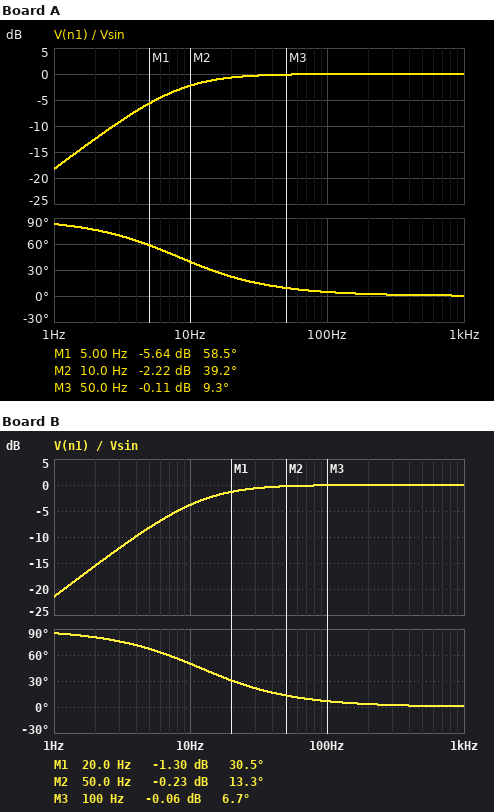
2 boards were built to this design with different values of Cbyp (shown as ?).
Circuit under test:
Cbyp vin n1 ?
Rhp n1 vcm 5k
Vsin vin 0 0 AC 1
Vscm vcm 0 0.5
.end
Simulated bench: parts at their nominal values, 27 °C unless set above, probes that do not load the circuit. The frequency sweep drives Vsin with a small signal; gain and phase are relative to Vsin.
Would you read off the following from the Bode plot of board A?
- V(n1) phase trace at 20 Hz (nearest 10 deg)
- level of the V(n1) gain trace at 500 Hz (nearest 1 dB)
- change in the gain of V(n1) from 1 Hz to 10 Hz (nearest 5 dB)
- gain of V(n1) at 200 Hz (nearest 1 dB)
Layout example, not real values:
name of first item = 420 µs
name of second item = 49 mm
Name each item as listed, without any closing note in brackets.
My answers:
V(n1) phase trace at 20 Hz = 20 deg
level of the V(n1) gain trace at 500 Hz = 0 dB
change in the gain of V(n1) from 1 Hz to 10 Hz = 15 dB
gain of V(n1) at 200 Hz = 0 dB
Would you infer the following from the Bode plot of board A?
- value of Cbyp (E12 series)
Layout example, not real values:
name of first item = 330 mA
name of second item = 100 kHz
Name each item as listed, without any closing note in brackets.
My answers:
value of Cbyp = 3.9 µF
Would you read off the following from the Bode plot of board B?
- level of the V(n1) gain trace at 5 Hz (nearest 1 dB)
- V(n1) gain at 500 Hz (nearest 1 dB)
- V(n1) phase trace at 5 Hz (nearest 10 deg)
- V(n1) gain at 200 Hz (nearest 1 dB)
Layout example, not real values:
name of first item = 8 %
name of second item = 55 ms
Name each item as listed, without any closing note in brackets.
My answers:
level of the V(n1) gain trace at 5 Hz = -8 dB
V(n1) gain at 500 Hz = 0 dB
V(n1) phase trace at 5 Hz = 70 deg
V(n1) gain at 200 Hz = 0 dB
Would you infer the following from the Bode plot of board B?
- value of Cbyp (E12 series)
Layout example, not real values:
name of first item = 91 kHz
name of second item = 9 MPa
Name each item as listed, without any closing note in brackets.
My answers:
value of Cbyp = 2.7 µF
